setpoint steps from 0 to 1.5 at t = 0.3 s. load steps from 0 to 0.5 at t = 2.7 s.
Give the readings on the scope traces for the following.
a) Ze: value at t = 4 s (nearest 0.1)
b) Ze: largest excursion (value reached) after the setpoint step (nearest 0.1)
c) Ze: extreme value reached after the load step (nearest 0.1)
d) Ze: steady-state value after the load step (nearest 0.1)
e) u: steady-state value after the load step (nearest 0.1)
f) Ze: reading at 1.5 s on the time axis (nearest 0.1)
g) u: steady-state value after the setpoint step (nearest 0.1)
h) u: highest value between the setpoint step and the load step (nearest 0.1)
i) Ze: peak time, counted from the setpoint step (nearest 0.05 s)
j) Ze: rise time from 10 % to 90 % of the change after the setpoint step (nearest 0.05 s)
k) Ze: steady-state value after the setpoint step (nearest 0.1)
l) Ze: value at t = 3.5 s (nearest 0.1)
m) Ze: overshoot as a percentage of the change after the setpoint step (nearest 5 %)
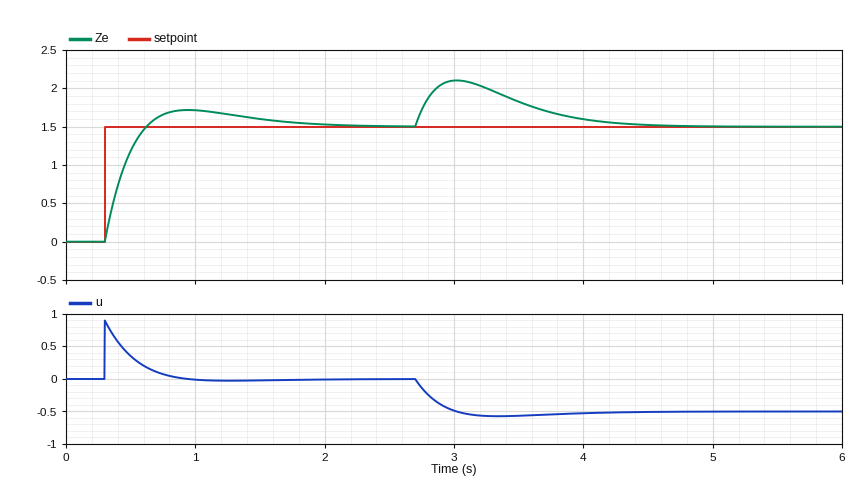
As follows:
1.6
1.7
2.1
1.5
-0.5
1.6
0.0
0.9
0.65 s
0.25 s
1.5
1.8
15 %
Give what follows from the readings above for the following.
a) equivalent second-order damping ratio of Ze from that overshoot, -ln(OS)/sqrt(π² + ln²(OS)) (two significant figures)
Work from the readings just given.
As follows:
0.52
